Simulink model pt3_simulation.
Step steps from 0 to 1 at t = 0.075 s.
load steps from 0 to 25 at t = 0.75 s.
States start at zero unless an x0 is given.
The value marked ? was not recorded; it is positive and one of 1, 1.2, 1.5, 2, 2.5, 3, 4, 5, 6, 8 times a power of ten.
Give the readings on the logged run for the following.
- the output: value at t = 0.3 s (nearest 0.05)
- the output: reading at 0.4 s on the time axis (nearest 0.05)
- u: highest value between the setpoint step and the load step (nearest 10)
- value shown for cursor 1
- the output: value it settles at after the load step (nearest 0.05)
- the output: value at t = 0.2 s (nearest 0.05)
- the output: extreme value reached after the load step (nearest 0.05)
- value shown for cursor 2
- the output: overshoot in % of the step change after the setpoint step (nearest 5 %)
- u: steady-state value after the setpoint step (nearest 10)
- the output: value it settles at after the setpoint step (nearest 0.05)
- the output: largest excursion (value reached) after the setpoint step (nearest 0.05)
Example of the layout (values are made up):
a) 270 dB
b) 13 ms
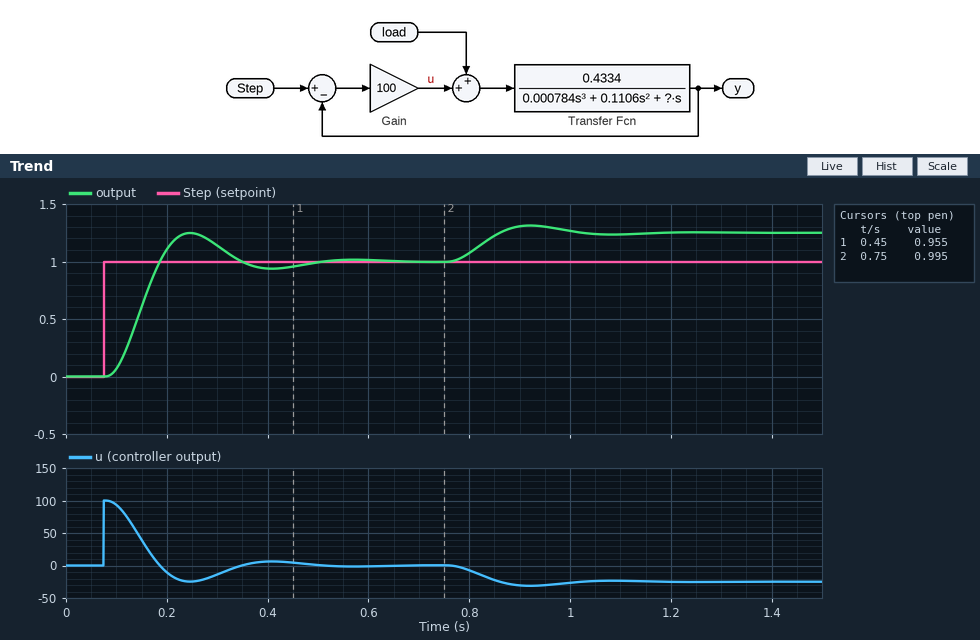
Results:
a) 1.15
b) 0.95
c) 100
d) 0.955
e) 1.25
f) 1.10
g) 1.30
h) 0.995
i) 25 %
j) 0
k) 1.00
l) 1.25
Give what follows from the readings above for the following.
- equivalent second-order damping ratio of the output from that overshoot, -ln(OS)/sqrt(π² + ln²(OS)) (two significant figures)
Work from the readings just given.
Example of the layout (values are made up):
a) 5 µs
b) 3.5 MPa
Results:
a) 0.40
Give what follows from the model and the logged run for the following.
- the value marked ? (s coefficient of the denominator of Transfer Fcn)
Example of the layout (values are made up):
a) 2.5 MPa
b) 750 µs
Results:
a) 2
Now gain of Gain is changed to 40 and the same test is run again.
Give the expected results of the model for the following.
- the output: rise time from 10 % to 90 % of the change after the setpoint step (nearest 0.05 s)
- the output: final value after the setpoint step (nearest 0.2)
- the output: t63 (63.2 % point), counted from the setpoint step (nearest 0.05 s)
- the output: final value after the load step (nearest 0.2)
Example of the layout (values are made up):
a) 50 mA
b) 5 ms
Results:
a) 0.15 s
b) 1.0
c) 0.15 s
d) 1.6
